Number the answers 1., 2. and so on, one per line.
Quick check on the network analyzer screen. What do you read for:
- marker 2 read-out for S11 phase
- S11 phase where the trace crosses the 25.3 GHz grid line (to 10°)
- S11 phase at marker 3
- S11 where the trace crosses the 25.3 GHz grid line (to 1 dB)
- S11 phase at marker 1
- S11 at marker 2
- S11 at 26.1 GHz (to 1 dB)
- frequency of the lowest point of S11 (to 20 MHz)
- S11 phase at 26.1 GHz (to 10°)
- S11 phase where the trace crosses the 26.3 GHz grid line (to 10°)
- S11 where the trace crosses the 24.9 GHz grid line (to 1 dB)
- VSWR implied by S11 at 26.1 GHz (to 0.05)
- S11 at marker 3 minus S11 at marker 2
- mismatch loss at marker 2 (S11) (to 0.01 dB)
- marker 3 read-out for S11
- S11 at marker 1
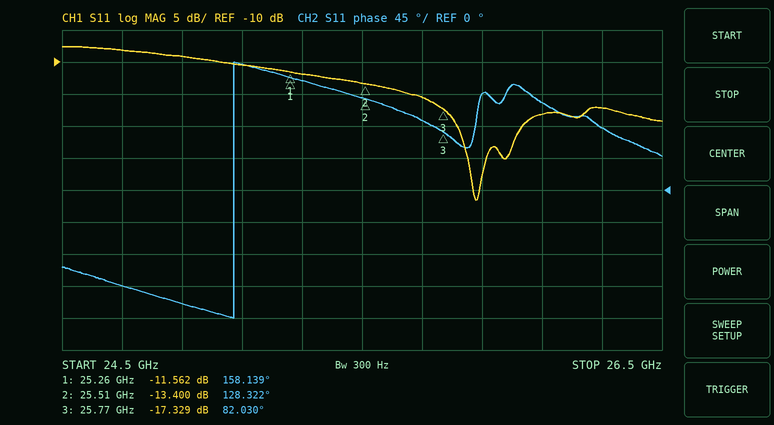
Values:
1. 128.322°
2. 150°
3. 82.030°
4. -12 dB
5. 158.139°
6. -13.400 dB
7. -18 dB
8. 25.88 GHz
9. 120°
10. 90°
11. -9 dB
12. 1.30
13. -3.929 dB
14. 0.20 dB
15. -17.329 dB
16. -11.562 dB
